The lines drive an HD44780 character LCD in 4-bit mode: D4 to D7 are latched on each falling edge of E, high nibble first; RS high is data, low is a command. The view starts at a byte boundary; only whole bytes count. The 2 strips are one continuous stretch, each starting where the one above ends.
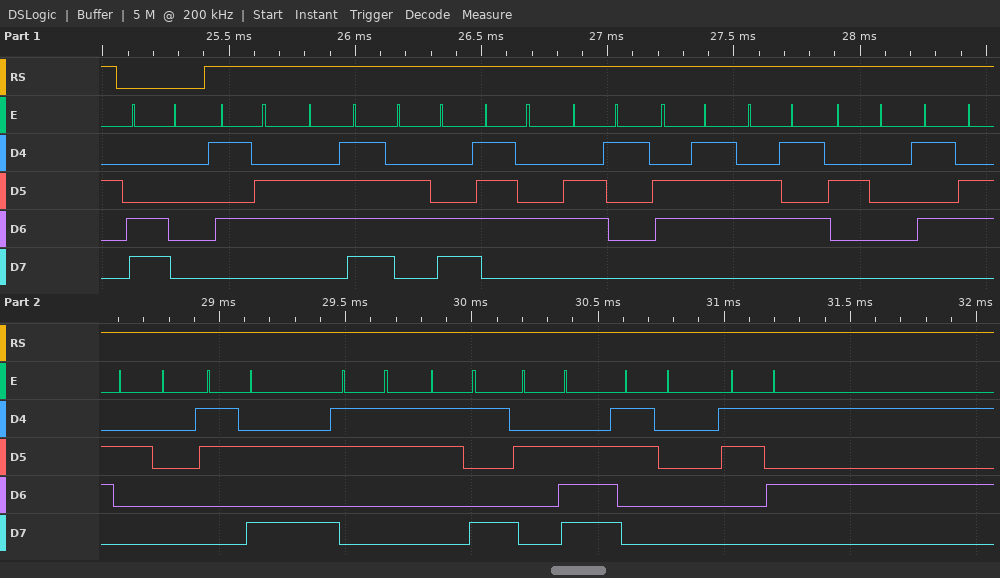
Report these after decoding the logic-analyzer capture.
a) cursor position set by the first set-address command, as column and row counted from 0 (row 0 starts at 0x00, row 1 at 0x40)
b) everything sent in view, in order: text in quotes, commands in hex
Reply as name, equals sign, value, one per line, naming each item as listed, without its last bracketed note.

cursor position set by the first set-address command, as column and row counted from 0 = column 0, row 1
everything sent in view, in order: text in quotes, commands in hex = 0xC0 "Voltage V :39.05"
